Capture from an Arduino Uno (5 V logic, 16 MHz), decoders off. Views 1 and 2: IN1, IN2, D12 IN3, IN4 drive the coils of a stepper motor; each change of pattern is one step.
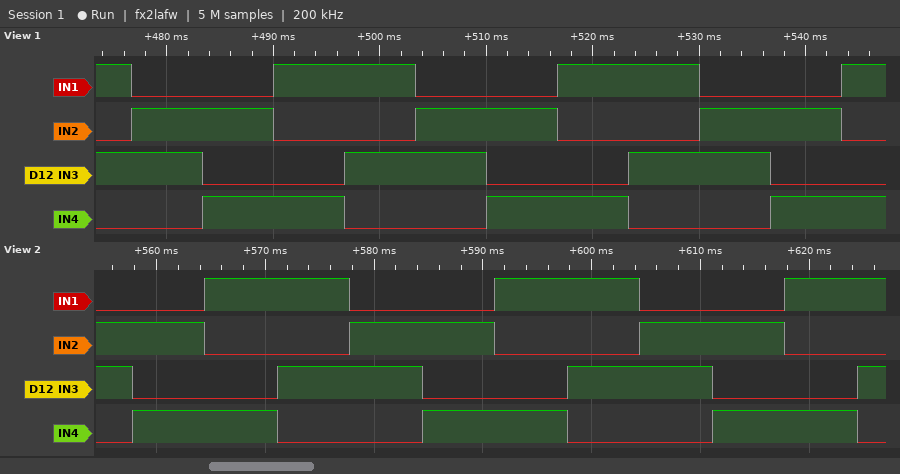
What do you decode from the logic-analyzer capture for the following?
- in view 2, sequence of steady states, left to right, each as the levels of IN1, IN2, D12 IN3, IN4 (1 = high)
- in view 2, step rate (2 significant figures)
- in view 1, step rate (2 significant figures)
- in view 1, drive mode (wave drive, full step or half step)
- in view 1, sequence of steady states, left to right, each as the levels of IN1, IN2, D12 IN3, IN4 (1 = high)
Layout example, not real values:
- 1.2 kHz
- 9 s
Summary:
- 0110 0101 1001 1010 0110 0101 1001 1010 0110 0101 1001 1010
- 150 steps/s
- 150 steps/s
- full step
- 1010 0110 0101 1001 1010 0110 0101 1001 1010 0110 0101 1001
